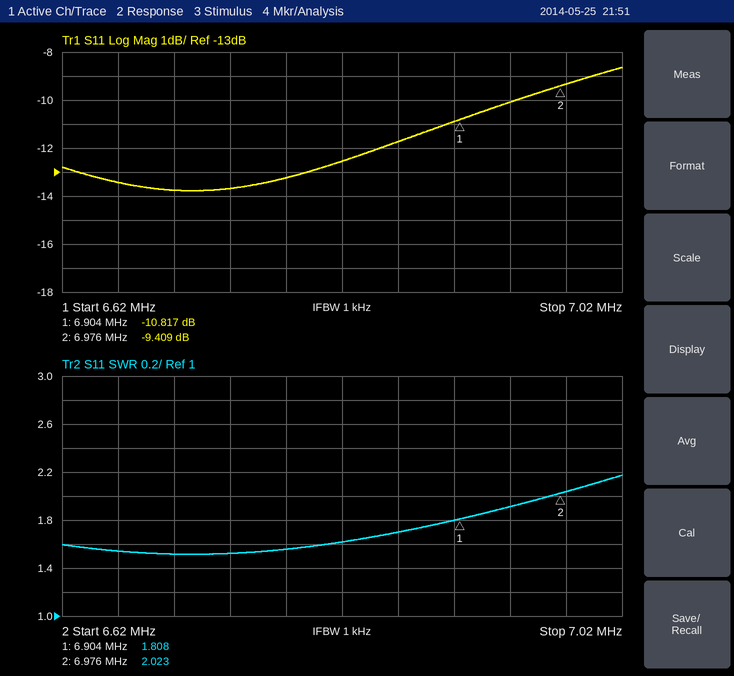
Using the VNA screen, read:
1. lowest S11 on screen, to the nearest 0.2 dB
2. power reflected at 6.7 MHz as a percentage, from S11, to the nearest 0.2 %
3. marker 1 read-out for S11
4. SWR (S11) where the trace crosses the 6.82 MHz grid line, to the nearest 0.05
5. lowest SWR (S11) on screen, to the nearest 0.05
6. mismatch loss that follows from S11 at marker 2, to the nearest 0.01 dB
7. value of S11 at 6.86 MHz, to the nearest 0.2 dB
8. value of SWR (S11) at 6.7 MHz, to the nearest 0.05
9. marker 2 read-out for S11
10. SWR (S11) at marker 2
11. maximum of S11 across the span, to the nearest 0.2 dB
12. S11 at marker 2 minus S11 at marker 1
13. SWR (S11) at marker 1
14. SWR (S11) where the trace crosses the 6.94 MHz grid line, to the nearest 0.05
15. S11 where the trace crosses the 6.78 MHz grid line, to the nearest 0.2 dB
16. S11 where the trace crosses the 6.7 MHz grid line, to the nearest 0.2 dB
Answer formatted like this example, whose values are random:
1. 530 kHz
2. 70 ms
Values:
1. -13.8 dB
2. 4.2 %
3. -10.817 dB
4. 1.60
5. 1.50
6. 0.53 dB
7. -11.8 dB
8. 1.50
9. -9.409 dB
10. 2.023
11. -8.6 dB
12. 1.408 dB
13. 1.808
14. 1.90
15. -13.2 dB
16. -13.8 dB
